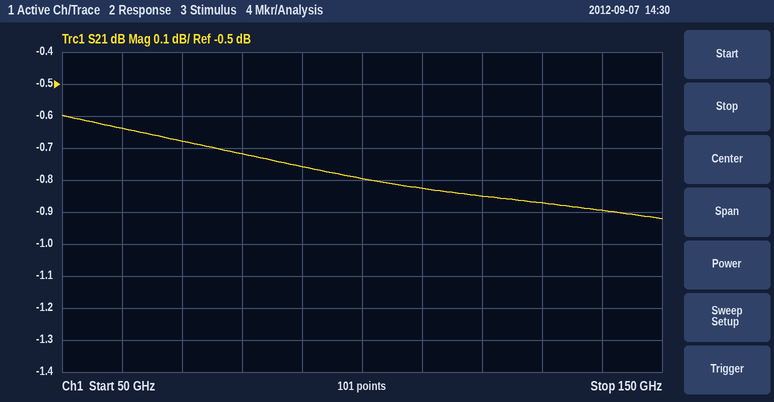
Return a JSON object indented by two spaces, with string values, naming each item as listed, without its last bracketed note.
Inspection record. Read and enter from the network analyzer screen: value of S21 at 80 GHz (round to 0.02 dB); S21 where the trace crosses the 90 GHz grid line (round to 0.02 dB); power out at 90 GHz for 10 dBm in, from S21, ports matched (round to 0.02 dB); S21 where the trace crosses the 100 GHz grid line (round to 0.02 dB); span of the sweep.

{
  "value of S21 at 80 GHz": "-0.72 dB",
  "S21 where the trace crosses the 90 GHz grid line": "-0.76 dB",
  "power out at 90 GHz for 10 dBm in, from S21, ports matched": "9.24 dBm",
  "S21 where the trace crosses the 100 GHz grid line": "-0.80 dB",
  "span of the sweep": "100 GHz"
}
